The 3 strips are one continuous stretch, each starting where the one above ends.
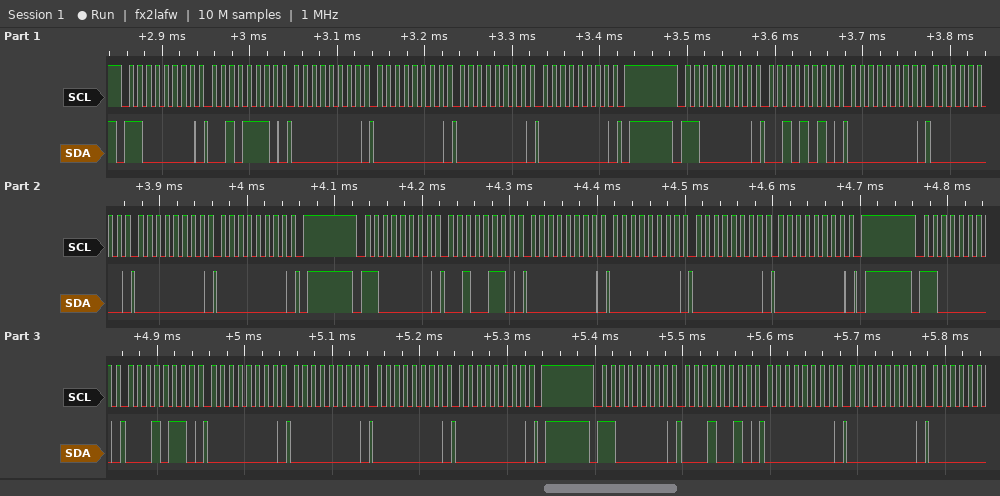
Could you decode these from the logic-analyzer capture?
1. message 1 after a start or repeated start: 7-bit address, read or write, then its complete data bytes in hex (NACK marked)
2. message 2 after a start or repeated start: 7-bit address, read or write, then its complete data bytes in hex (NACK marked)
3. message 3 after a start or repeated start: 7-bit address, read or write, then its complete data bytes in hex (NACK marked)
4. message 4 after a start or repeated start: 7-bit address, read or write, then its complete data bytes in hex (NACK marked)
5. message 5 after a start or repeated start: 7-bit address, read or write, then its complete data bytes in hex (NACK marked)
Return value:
0x60 write: 2E 00 00 00 00
0x60 write: 2A 00 00 00 00
0x60 write: 26 00 00 00 00
0x60 write: 16 00 00 00 00
0x60 write: 12 00 00
